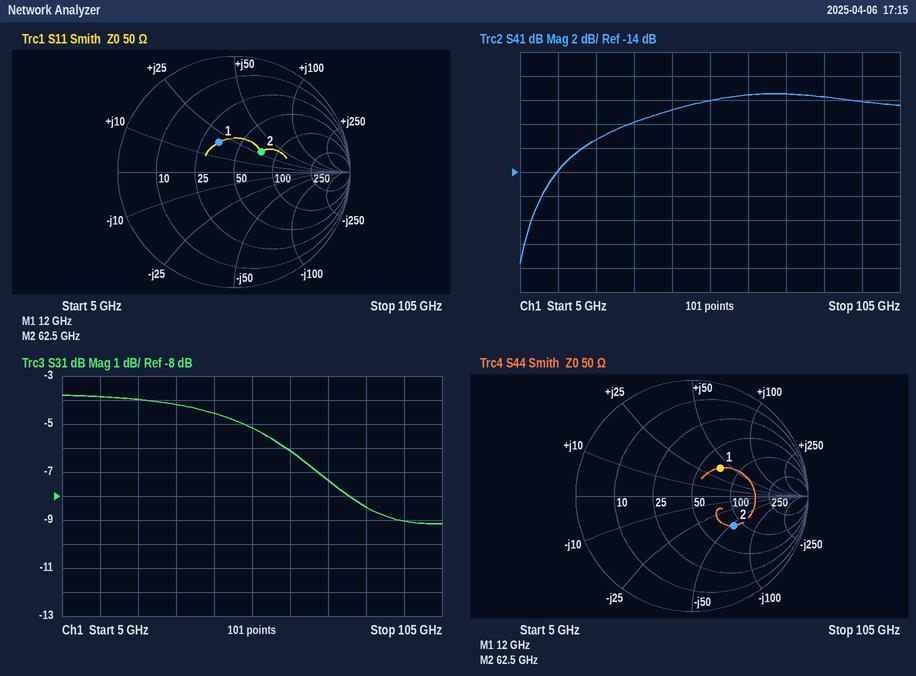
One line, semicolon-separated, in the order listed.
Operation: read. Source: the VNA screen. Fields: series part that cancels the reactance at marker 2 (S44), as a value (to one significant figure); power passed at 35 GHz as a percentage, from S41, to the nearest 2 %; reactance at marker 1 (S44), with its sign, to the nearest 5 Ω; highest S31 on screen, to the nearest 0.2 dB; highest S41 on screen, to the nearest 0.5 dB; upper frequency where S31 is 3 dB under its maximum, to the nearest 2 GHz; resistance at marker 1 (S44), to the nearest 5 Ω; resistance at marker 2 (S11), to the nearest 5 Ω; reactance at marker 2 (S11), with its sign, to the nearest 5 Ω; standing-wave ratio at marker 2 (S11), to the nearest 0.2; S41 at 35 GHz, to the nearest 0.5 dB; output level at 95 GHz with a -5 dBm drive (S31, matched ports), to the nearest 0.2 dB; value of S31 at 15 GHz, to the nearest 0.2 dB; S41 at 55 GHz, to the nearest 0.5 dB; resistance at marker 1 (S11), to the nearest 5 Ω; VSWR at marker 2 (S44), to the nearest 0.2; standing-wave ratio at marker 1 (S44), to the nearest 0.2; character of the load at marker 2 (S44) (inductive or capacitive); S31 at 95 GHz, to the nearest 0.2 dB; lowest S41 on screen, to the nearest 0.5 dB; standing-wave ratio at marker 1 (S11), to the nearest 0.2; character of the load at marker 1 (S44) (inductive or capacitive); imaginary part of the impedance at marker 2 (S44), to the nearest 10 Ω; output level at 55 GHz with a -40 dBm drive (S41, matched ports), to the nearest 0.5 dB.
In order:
100 pH; 10 %; +40 Ω; -3.8 dB; -7.5 dB; 70 GHz; 70 Ω; 75 Ω; +30 Ω; 1.8; -10.0 dB; -14.0 dBm; -3.8 dB; -8.0 dB; 35 Ω; 2.6; 2.0; capacitive; -9.0 dB; -21.5 dB; 1.8; inductive; -50 Ω; -48.0 dBm
